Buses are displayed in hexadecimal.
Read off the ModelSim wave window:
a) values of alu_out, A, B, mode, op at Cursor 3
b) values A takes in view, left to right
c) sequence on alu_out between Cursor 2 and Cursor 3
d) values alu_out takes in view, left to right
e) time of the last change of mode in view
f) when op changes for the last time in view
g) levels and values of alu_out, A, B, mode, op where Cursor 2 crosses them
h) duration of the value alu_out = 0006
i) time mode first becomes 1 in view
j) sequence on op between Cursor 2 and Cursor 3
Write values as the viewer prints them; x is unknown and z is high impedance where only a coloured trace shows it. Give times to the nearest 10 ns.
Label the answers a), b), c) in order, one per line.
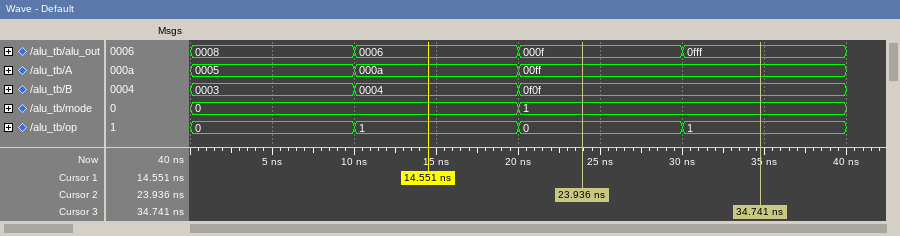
a) alu_out=0fff, A=00ff, B=0f0f, mode=1, op=1
b) 0005, 000a, 00ff
c) 000f, 0fff
d) 0008, 0006, 000f, 0fff
e) 20 ns
f) 30 ns
g) alu_out=000f, A=00ff, B=0f0f, mode=1, op=0
h) 10 ns
i) 20 ns
j) 0, 1
